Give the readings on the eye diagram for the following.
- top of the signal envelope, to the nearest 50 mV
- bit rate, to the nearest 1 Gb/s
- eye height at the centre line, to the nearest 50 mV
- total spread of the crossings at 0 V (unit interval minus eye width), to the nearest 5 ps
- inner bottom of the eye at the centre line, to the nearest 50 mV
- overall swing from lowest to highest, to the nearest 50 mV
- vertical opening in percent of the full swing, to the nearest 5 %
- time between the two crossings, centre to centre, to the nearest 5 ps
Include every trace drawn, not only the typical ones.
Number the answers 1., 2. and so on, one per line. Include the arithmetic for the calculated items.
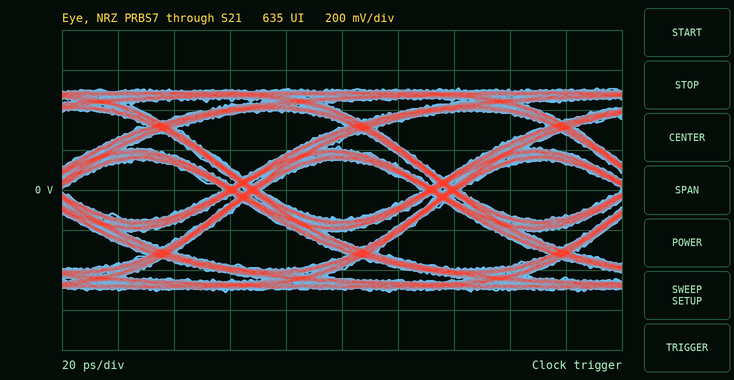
1. 500 mV
2. 14 Gb/s
3. 300 mV
4. 15 ps
5. -150 mV
6. 1.00 V
7. 300 mV / 1.00 V ≈ 30 %
8. 70 ps
